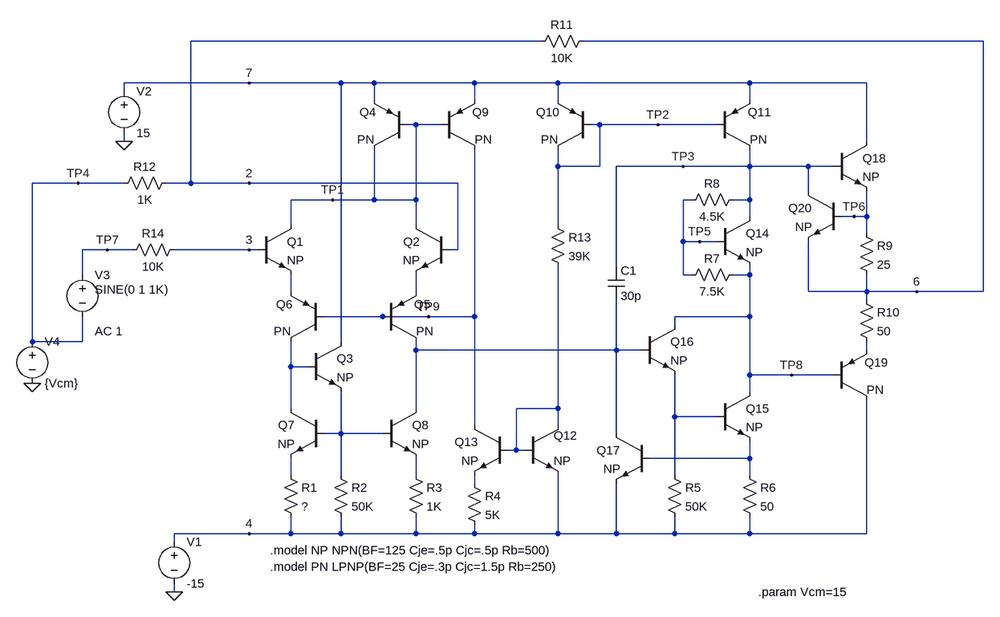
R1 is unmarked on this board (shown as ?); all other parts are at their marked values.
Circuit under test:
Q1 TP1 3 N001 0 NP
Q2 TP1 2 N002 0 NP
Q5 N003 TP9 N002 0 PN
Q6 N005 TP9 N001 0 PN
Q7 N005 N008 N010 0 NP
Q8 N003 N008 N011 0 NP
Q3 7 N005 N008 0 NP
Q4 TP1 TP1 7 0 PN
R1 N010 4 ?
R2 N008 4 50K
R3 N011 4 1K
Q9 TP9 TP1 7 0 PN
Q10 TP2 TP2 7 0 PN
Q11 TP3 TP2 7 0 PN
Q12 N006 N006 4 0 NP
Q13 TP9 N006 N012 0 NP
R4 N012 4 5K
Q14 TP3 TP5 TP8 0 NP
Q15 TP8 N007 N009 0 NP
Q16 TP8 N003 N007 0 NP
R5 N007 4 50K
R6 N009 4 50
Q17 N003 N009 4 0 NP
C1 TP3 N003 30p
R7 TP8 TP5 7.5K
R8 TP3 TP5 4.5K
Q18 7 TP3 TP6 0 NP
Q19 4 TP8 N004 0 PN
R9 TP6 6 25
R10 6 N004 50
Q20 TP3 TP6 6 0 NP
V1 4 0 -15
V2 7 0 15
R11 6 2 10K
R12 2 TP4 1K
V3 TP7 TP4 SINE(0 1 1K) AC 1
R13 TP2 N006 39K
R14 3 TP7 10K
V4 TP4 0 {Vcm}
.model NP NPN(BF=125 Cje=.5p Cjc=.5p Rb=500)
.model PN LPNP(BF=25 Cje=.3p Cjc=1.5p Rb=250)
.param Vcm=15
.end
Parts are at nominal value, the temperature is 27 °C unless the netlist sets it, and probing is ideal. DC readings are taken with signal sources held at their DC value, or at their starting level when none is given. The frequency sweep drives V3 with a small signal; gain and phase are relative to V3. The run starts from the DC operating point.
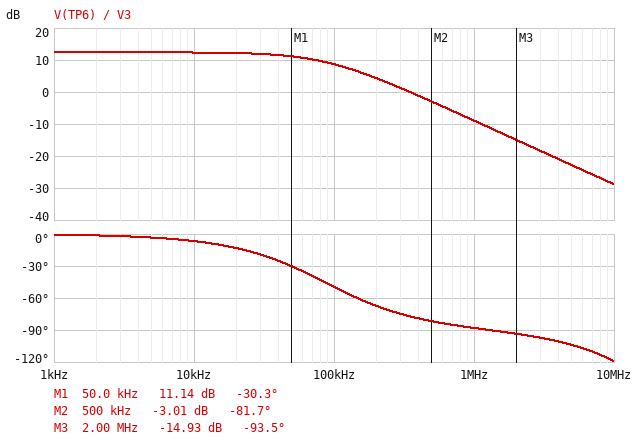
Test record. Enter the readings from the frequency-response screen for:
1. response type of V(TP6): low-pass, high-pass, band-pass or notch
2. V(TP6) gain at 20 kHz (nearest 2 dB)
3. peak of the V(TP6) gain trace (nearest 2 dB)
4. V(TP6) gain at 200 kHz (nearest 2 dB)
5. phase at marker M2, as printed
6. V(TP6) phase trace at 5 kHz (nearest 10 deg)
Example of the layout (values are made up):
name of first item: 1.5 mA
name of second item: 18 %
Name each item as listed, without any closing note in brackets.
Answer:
response type of V(TP6): low-pass, high-pass, band-pass or notch: low-pass
V(TP6) gain at 20 kHz: 12 dB
peak of the V(TP6) gain trace: 12 dB
V(TP6) gain at 200 kHz: 4 dB
phase at marker M2, as printed: -81.7 deg
V(TP6) phase trace at 5 kHz: 0 deg
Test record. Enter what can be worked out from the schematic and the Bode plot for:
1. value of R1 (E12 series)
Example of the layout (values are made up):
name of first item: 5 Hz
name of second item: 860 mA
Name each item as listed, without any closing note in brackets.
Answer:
value of R1: 330 Ω
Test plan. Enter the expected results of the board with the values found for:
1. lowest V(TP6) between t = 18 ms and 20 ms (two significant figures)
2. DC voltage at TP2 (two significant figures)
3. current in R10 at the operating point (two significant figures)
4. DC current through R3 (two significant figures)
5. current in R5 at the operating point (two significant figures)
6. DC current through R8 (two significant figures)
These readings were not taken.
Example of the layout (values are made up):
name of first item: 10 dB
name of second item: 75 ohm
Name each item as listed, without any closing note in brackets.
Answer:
lowest V(TP6) between t = 18 ms and 20 ms: 3.9 V
DC voltage at TP2: 14 V
current in R10 at the operating point: 51 µA
DC current through R3: 11 µA
current in R5 at the operating point: 15 µA
DC current through R8: 100 µA
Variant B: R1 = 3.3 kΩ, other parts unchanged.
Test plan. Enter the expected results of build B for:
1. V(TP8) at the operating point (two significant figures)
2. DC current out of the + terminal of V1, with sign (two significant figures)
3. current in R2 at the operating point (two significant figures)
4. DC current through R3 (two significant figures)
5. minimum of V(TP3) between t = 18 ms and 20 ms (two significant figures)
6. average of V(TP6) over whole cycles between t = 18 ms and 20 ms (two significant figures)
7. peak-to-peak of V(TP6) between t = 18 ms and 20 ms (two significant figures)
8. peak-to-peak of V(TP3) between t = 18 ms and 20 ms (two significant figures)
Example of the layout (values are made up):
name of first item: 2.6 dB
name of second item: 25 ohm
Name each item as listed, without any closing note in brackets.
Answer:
V(TP8) at the operating point: 15 V
DC current out of the + terminal of V1, with sign: -800 µA
current in R2 at the operating point: 14 µA
DC current through R3: 23 µA
minimum of V(TP3) between t = 18 ms and 20 ms: 4.7 V
average of V(TP6) over whole cycles between t = 18 ms and 20 ms: 12 V
peak-to-peak of V(TP6) between t = 18 ms and 20 ms: 11 V
peak-to-peak of V(TP3) between t = 18 ms and 20 ms: 10 V
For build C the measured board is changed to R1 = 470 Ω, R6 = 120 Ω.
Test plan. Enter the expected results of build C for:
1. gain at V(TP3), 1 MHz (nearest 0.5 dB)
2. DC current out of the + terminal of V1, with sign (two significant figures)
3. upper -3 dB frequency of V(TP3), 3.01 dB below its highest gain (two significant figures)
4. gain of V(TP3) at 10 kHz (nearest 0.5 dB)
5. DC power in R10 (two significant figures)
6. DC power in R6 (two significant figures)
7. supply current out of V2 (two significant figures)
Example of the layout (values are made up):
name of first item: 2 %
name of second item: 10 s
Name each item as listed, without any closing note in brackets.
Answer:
gain at V(TP3), 1 MHz: -18.5 dB
DC current out of the + terminal of V1, with sign: -1.1 mA
upper -3 dB frequency of V(TP3), 3.01 dB below its highest gain: 81 kHz
gain of V(TP3) at 10 kHz: 3.0 dB
DC power in R10: 110 nW
DC power in R6: 8.6 µW
supply current out of V2: 1.1 mA
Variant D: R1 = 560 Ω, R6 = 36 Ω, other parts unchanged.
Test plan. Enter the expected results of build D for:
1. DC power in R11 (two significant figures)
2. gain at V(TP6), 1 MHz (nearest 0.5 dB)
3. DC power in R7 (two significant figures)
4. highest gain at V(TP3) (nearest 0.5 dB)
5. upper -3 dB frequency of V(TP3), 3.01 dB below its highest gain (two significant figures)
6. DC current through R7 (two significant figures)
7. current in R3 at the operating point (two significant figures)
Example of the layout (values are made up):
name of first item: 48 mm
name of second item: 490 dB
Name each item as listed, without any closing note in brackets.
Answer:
DC power in R11: 21 µW
gain at V(TP6), 1 MHz: -5.0 dB
DC power in R7: 69 µW
highest gain at V(TP3): 1.0 dB
upper -3 dB frequency of V(TP3), 3.01 dB below its highest gain: 120 kHz
DC current through R7: 96 µA
current in R3 at the operating point: 12 µA
